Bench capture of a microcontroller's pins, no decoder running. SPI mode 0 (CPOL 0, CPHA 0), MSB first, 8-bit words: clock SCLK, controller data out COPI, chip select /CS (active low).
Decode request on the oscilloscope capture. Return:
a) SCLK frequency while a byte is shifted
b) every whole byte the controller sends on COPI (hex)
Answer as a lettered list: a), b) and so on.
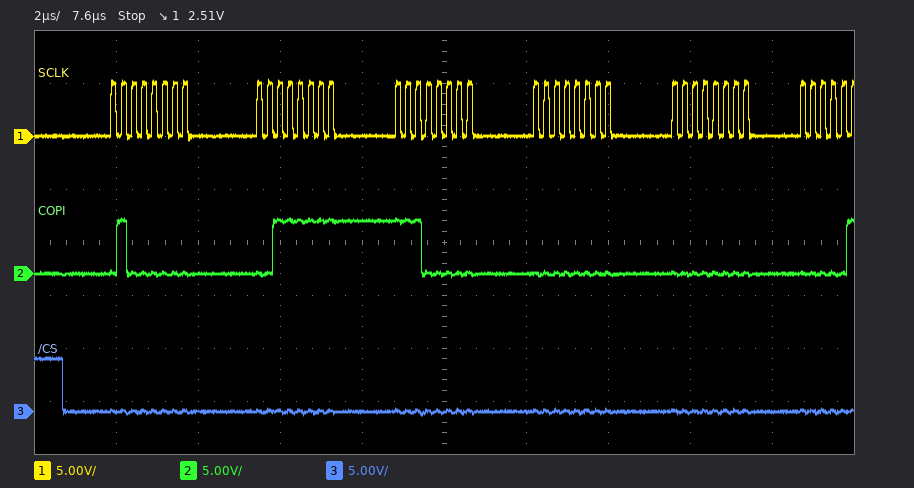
a) 4 MHz
b) 40 3F E0 00 00
